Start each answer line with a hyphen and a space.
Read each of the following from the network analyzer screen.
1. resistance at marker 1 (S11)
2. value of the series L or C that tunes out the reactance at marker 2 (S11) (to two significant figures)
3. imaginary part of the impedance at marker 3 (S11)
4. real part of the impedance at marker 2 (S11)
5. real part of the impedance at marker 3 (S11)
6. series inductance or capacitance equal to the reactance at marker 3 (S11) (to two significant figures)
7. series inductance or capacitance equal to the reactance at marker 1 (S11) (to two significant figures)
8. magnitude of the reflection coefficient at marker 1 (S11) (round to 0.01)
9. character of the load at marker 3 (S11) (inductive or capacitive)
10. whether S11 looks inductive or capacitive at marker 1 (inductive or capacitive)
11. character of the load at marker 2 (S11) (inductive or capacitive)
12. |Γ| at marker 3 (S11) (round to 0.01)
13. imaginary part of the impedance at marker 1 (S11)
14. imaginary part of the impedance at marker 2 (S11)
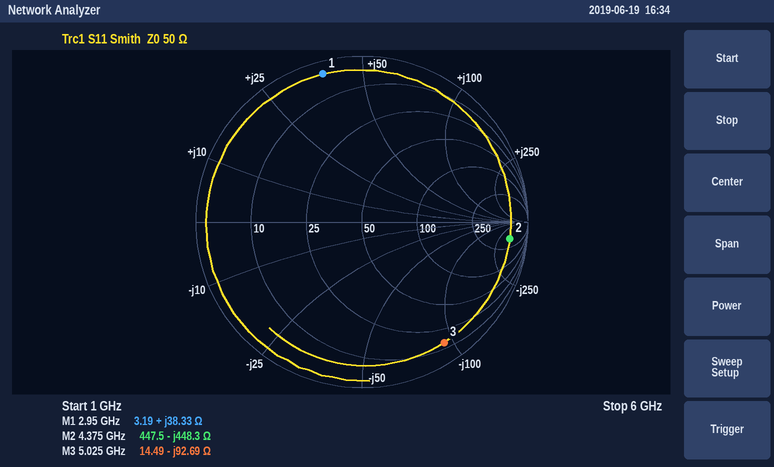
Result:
- 3.19 Ω
- 16 nH
- -92.69 Ω
- 447.5 Ω
- 14.49 Ω
- 340 fF
- 2.1 nH
- 0.92
- capacitive
- inductive
- capacitive
- 0.88
- +38.33 Ω
- -448.3 Ω
